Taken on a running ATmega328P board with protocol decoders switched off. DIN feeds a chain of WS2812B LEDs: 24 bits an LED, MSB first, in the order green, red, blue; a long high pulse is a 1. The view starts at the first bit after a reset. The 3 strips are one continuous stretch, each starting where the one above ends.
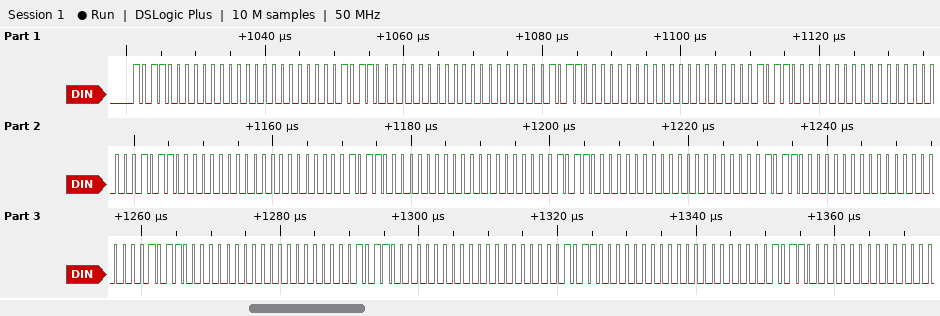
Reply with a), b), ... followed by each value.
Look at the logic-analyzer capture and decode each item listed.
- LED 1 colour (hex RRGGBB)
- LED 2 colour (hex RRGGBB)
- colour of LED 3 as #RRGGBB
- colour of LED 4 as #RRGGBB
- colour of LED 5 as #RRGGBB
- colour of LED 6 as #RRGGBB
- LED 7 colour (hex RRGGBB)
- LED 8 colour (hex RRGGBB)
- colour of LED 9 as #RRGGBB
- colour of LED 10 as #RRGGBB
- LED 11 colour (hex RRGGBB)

a) #00B000
b) #00B000
c) #00B000
d) #00B000
e) #00B000
f) #00B000
g) #00B000
h) #00B000
i) #00B000
j) #00B000
k) #00B000
